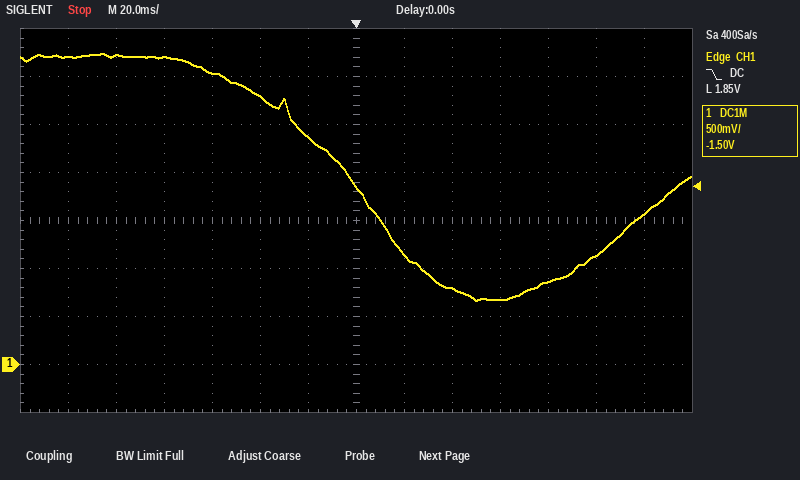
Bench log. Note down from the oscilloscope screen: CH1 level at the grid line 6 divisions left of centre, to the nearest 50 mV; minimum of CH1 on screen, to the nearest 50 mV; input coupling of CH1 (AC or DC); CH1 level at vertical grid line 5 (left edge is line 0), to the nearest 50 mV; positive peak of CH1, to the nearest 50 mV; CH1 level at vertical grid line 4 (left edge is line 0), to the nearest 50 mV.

3.20 V
650 mV
DC
2.80 V
3.25 V
3.05 V
